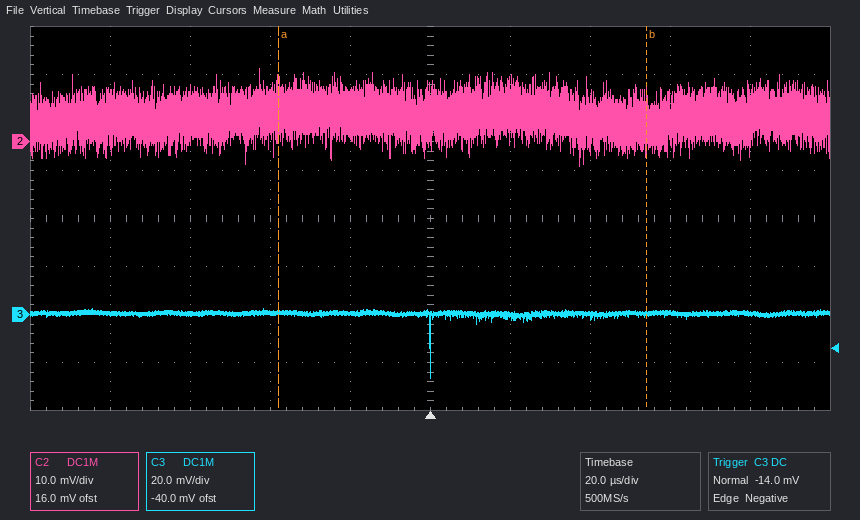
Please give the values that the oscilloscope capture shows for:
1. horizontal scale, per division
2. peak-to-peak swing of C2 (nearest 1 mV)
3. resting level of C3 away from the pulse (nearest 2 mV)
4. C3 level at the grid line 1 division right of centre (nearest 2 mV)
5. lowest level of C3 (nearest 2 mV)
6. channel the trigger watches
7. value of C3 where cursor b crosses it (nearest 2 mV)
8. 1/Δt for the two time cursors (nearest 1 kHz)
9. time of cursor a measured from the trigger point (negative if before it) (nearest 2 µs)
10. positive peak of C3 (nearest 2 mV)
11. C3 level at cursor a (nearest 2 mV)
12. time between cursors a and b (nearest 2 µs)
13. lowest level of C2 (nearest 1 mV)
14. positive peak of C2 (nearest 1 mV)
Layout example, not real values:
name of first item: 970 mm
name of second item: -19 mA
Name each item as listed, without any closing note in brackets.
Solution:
horizontal scale, per division: 20 µs
peak-to-peak swing of C2: 20 mV
resting level of C3 away from the pulse: 0 mV
C3 level at the grid line 1 division right of centre: 0 mV
lowest level of C3: -26 mV
channel the trigger watches: C3
value of C3 where cursor b crosses it: 0 mV
1/Δt for the two time cursors: 11 kHz
time of cursor a measured from the trigger point (negative if before it): -38 µs
positive peak of C3: 2 mV
C3 level at cursor a: 0 mV
time between cursors a and b: 92 µs
lowest level of C2: -5 mV
positive peak of C2: 15 mV
